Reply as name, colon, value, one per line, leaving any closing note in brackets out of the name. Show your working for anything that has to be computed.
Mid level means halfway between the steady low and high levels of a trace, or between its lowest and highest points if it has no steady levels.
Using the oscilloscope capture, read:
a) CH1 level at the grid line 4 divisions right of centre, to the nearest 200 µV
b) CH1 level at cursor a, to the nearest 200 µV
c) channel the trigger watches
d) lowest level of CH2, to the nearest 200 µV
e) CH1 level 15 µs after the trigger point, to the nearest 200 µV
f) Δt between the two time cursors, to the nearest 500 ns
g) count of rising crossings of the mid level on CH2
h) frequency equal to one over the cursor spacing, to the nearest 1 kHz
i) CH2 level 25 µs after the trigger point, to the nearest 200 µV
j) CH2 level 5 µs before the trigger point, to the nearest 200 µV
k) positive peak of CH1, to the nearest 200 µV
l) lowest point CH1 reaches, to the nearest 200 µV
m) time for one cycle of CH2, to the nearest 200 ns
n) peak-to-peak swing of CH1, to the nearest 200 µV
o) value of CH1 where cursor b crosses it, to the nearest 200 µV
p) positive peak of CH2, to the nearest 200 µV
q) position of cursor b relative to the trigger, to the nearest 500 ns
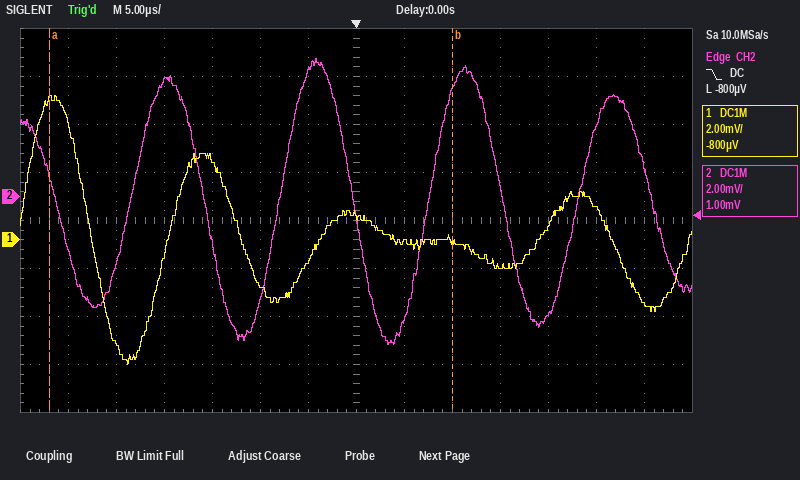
CH1 level at the grid line 4 divisions right of centre, to the nearest 200 µV: 600 µV
CH1 level at cursor a, to the nearest 200 µV: 5.8 mV
channel the trigger watches: CH2
lowest level of CH2, to the nearest 200 µV: -6.2 mV
CH1 level 15 µs after the trigger point, to the nearest 200 µV: -1.2 mV
Δt between the two time cursors, to the nearest 500 ns: 42.0 µs
count of rising crossings of the mid level on CH2: 4
frequency equal to one over the cursor spacing, to the nearest 1 kHz: 1 / 42.0 µs ≈ 24 kHz
CH2 level 25 µs after the trigger point, to the nearest 200 µV: 3.0 mV
CH2 level 5 µs before the trigger point, to the nearest 200 µV: 5.2 mV
positive peak of CH1, to the nearest 200 µV: 6.0 mV
lowest point CH1 reaches, to the nearest 200 µV: -5.2 mV
time for one cycle of CH2, to the nearest 200 ns: 15.6 µs
peak-to-peak swing of CH1, to the nearest 200 µV: 6.0 mV − (-5.2 mV) = 11.2 mV
value of CH1 where cursor b crosses it, to the nearest 200 µV: 0.0 mV
positive peak of CH2, to the nearest 200 µV: 5.8 mV
position of cursor b relative to the trigger, to the nearest 500 ns: +10.0 µs
